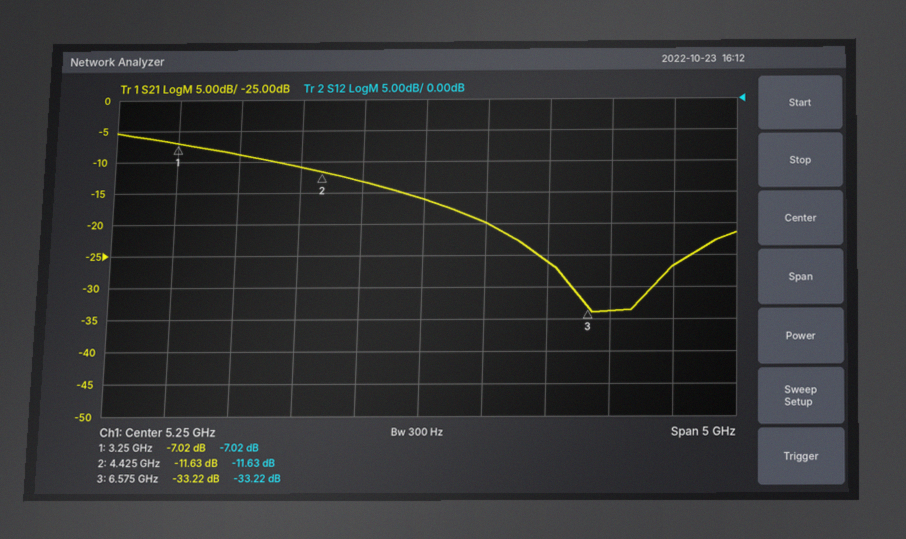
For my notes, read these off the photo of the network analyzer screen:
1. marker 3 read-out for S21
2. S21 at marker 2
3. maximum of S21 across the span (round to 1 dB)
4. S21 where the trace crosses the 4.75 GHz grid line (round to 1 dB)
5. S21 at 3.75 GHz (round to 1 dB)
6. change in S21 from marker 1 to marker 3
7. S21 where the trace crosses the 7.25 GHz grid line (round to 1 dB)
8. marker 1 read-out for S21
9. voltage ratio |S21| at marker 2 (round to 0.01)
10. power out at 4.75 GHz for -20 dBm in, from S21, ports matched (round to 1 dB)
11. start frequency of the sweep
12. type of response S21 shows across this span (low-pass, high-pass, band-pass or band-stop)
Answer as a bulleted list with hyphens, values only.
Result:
- -33.22 dB
- -11.63 dB
- -5 dB
- -13 dB
- -9 dB
- -26.20 dB
- -27 dB
- -7.02 dB
- 0.26
- -33 dBm
- 2.75 GHz
- low-pass
